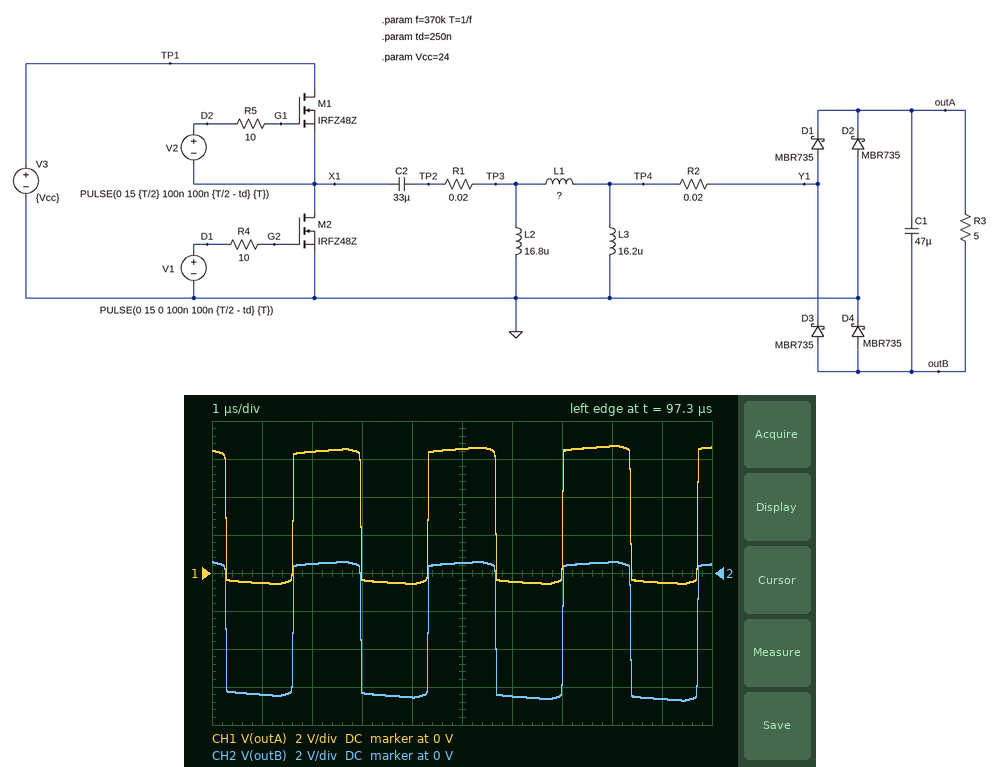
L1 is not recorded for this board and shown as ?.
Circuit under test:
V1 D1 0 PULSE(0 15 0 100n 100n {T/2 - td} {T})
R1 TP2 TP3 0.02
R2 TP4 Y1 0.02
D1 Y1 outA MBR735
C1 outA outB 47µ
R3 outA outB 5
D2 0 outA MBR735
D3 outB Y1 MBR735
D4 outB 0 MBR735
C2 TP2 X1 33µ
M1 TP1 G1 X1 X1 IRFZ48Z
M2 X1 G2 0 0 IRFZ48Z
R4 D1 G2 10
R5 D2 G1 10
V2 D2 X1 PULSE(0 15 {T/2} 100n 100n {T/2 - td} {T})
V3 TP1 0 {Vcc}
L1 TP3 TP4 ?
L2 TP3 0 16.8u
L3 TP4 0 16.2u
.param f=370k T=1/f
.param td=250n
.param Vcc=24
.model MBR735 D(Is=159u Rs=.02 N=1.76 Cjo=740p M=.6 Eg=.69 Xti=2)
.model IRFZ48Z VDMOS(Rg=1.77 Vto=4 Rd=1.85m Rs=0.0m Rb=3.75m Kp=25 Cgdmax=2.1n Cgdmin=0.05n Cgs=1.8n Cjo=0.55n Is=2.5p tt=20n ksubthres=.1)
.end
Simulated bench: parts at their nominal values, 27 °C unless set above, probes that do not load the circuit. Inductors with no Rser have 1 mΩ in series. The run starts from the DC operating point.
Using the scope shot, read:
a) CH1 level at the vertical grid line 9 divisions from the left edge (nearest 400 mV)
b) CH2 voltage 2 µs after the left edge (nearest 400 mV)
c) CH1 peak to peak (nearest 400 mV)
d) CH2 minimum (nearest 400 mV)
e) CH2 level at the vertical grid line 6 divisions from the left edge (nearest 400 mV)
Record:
-400 mV
400 mV
7.2 V
-6.8 V
-6.4 V
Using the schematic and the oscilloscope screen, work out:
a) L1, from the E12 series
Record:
1 µH
